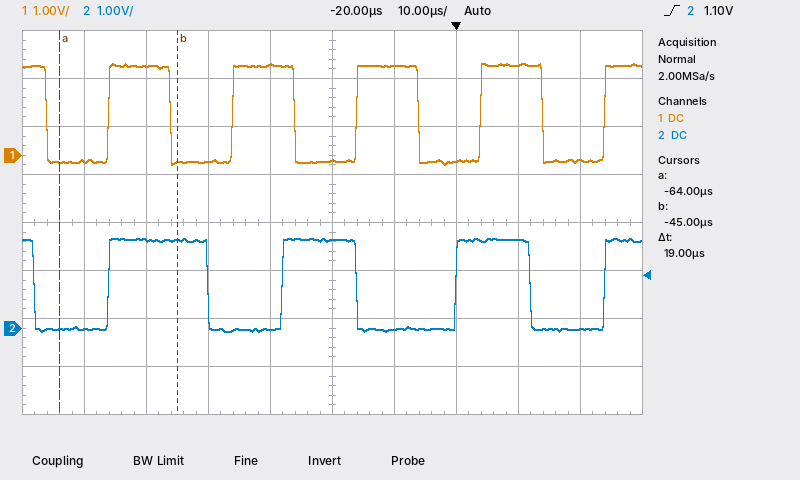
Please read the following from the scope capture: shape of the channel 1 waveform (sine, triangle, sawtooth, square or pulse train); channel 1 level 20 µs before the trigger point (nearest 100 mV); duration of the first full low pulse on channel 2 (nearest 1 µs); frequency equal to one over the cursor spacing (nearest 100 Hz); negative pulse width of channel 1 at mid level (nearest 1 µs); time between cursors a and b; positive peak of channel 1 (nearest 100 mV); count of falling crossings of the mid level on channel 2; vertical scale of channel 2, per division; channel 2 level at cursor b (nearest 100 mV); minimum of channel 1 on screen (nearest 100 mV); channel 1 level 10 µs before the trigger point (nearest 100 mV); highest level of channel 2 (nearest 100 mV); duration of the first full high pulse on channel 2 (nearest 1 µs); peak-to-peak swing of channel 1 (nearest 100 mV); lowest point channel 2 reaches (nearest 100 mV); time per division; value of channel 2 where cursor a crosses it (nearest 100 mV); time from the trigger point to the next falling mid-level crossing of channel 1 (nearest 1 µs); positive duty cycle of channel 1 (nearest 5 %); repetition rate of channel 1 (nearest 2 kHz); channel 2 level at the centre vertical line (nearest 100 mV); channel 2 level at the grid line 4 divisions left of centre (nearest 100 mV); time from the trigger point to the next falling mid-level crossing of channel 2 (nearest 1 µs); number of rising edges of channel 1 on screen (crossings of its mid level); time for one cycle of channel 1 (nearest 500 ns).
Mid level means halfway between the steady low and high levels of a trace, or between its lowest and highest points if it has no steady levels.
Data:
square
-100 mV
12 µs
52.6 kHz
10 µs
19 µs
1.9 V
4
1 V
1.8 V
-200 mV
1.9 V
1.9 V
16 µs
2.1 V
-100 mV
10 µs
0.0 V
14 µs
50 %
50 kHz
1.8 V
0.0 V
12 µs
5
20.0 µs
